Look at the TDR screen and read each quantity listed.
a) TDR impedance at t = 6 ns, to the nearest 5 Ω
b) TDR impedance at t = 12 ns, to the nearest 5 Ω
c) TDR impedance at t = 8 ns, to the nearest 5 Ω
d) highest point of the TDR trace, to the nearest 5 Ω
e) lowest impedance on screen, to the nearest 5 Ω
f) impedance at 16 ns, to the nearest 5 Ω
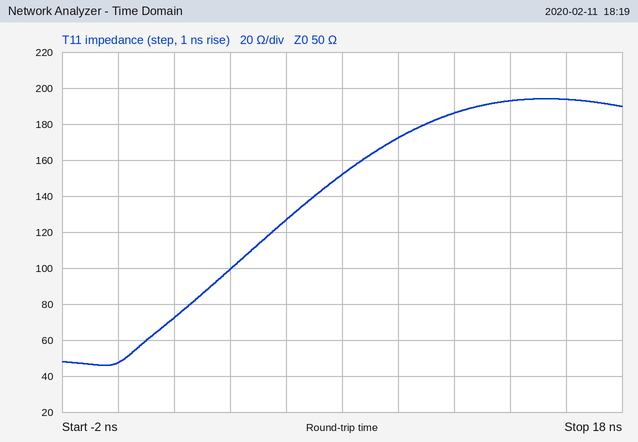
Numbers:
125 Ω
185 Ω
150 Ω
195 Ω
45 Ω
195 Ω
